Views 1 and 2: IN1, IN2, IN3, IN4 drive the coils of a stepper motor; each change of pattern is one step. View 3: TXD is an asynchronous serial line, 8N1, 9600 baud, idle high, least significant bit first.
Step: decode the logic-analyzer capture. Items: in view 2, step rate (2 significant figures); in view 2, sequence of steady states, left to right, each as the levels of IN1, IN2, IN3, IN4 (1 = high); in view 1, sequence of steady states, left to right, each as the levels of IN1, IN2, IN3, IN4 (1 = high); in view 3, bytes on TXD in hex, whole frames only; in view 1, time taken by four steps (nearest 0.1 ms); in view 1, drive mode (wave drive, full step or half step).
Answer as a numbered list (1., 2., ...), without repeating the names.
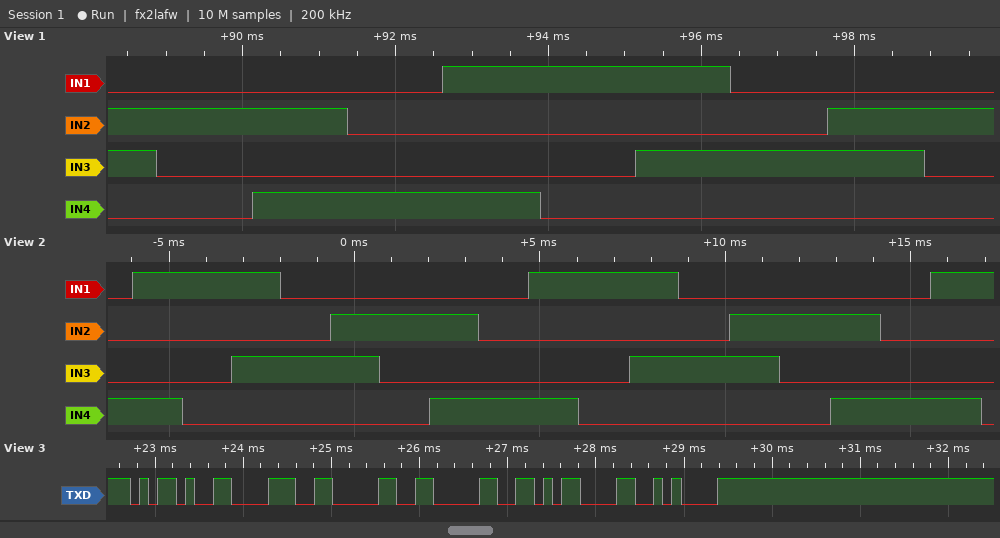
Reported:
1. 740 steps/s
2. 0001 1001 1000 1010 0010 0110 0100 0101 0001 1001 1000 1010 0010 0110 0100 0101 0001 1001 1000
3. 0110 0100 0101 0001 1001 1000 1010 0010 0110 0100
4. 2D 38 30 30 0D 0A
5. 5.0 ms
6. half step
